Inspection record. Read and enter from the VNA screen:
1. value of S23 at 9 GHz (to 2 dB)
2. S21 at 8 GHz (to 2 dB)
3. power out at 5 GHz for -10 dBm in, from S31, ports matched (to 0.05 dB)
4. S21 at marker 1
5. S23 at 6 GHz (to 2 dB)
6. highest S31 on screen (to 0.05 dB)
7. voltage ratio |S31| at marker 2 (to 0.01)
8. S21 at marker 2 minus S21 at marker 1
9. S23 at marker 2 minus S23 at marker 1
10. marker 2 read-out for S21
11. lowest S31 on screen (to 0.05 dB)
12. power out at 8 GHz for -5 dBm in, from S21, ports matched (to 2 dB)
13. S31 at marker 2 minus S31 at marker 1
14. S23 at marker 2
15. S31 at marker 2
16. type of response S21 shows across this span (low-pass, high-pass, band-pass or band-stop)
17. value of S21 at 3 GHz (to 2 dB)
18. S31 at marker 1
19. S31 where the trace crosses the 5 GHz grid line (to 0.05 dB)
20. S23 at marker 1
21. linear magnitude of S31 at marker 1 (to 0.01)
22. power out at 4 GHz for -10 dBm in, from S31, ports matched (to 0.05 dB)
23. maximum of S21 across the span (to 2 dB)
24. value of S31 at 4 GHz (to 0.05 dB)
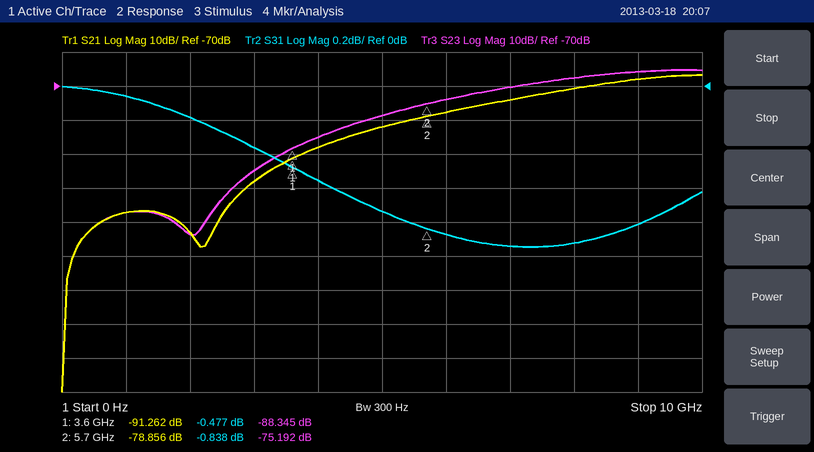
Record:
-66 dB
-70 dB
-10.75 dBm
-91.262 dB
-74 dB
0.00 dB
0.91
12.406 dB
13.153 dB
-78.856 dB
-0.95 dB
-76 dBm
-0.361 dB
-75.192 dB
-0.838 dB
high-pass
-98 dB
-0.477 dB
-0.75 dB
-88.345 dB
0.95
-10.55 dBm
-66 dB
-0.55 dB
